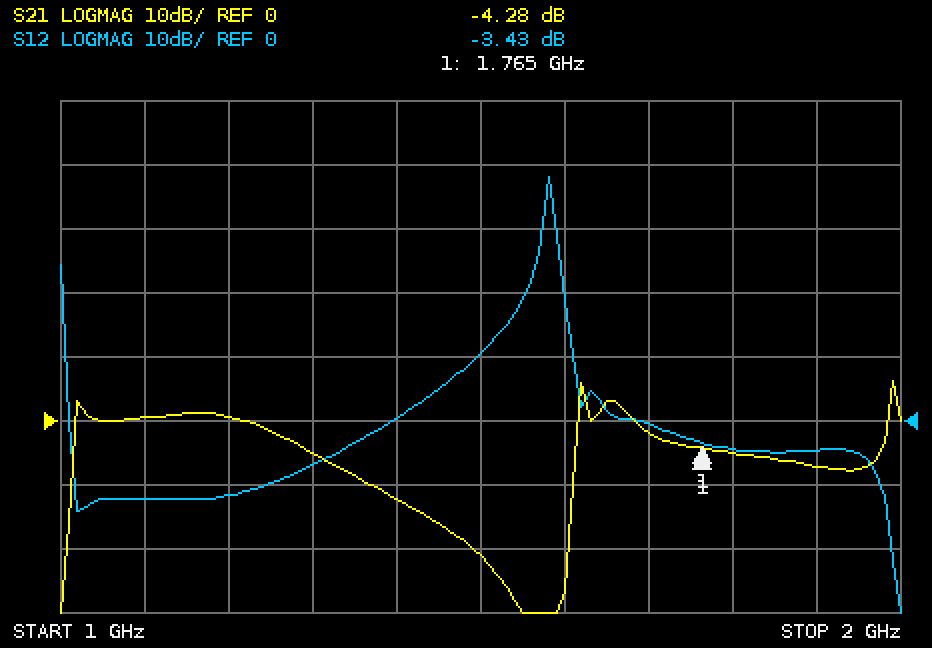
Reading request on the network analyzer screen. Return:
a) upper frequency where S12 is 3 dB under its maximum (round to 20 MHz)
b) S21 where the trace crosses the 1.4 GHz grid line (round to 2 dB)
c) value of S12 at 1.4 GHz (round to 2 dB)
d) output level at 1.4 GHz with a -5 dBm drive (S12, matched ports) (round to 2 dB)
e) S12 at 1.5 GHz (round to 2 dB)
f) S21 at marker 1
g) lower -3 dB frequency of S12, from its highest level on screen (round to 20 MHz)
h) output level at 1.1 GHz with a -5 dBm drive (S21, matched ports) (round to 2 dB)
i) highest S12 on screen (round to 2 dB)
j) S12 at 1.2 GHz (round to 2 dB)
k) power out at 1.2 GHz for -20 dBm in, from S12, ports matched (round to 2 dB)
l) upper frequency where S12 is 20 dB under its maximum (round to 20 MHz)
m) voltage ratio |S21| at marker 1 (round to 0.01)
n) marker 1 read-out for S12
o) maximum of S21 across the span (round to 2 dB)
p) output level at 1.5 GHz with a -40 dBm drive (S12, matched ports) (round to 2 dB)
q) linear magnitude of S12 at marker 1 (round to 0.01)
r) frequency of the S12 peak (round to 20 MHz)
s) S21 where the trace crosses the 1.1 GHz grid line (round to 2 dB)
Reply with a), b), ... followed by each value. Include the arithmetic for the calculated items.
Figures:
a) 1.58 GHz
b) -12 dB
c) 0 dB
d) -5 dBm + (0 dB) = -4 dBm
e) 10 dB
f) -4.28 dB
g) 1.58 GHz
h) -5 dBm + (0 dB) = -4 dBm
i) 38 dB
j) -12 dB
k) -20 dBm + (-12 dB) = -32 dBm
l) 1.60 GHz
m) 10^(-4.28/20) ≈ 0.61
n) -3.43 dB
o) 6 dB
p) -40 dBm + (10 dB) = -30 dBm
q) 10^(-3.43/20) ≈ 0.67
r) 1.58 GHz
s) 0 dB
